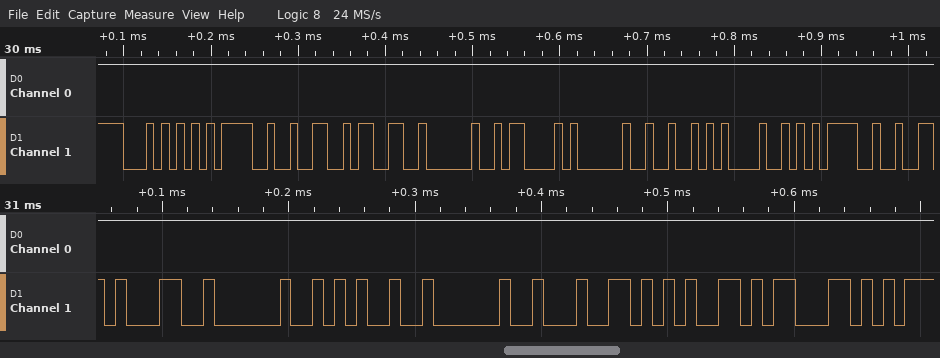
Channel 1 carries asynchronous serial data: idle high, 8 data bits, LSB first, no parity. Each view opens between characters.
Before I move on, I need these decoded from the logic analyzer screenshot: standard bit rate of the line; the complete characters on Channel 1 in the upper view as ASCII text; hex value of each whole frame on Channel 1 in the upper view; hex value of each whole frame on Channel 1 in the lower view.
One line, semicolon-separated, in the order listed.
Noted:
115200 baud; "T=23 C RH="; 54, 3D, 32, 33, 20, 43, 20, 52, 48, 3D; 31, 20, 25, 20, 64, 65, 63
